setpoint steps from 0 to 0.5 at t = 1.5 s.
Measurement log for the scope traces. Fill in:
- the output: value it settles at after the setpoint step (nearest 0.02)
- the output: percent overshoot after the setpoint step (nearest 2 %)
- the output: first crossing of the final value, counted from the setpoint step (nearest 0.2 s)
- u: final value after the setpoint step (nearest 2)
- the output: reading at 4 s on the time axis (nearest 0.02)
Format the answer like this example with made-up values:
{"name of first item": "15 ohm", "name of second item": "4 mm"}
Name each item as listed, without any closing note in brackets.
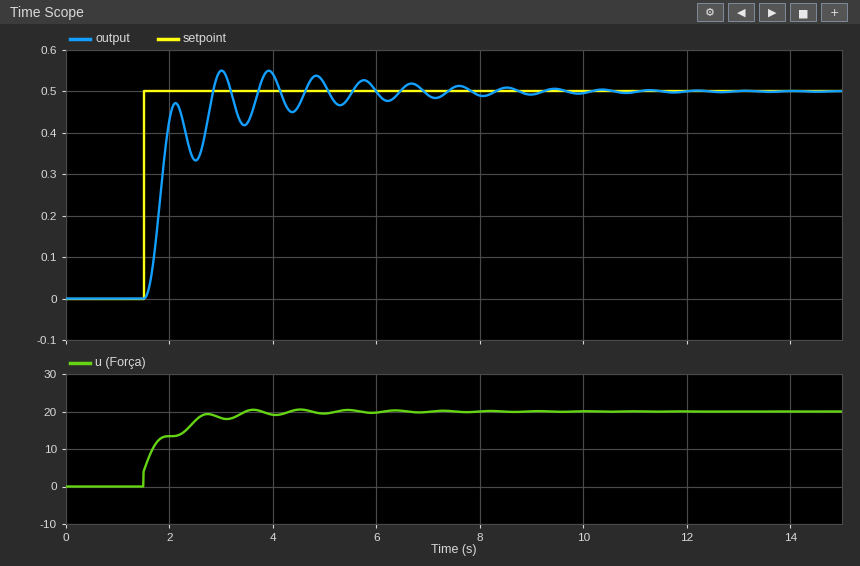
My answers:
{"the output: value it settles at after the setpoint step": "0.50", "the output: percent overshoot after the setpoint step": "10 %", "the output: first crossing of the final value, counted from the setpoint step": "1.4 s", "u: final value after the setpoint step": "20", "the output: reading at 4 s on the time axis": "0.54"}
